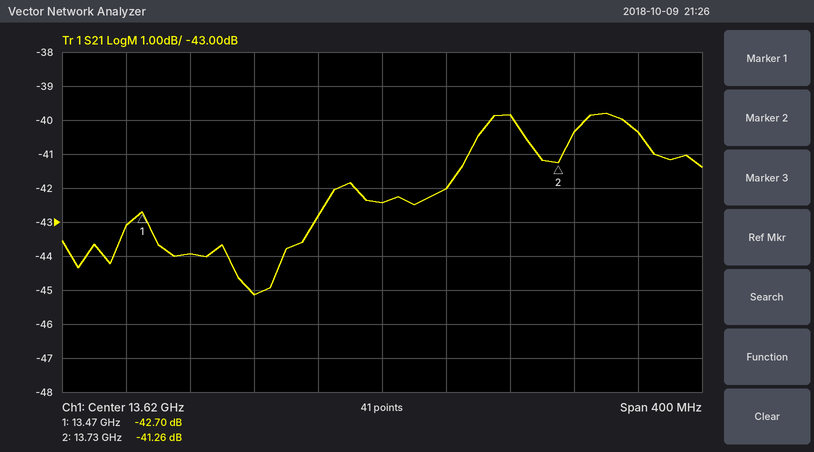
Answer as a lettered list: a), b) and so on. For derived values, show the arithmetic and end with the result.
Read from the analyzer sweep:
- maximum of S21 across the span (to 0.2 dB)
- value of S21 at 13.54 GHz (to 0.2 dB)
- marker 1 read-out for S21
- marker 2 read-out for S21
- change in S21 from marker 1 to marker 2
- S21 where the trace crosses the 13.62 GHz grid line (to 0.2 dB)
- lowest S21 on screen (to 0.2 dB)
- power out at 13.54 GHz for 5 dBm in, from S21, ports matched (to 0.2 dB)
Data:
a) -39.8 dB
b) -45.2 dB
c) -42.70 dB
d) -41.26 dB
e) -41.26 − (-42.7) = 1.44 dB
f) -42.4 dB
g) -45.2 dB
h) 5 dBm + (-45.2 dB) = -40.2 dBm
